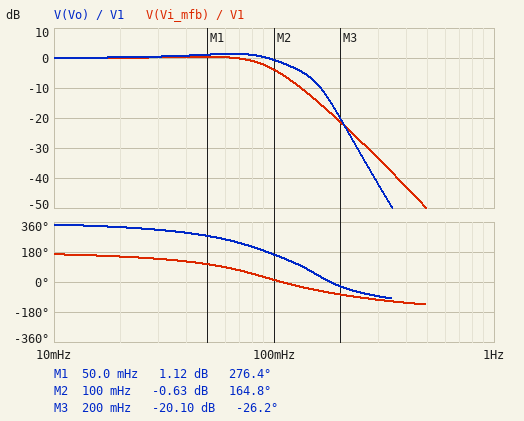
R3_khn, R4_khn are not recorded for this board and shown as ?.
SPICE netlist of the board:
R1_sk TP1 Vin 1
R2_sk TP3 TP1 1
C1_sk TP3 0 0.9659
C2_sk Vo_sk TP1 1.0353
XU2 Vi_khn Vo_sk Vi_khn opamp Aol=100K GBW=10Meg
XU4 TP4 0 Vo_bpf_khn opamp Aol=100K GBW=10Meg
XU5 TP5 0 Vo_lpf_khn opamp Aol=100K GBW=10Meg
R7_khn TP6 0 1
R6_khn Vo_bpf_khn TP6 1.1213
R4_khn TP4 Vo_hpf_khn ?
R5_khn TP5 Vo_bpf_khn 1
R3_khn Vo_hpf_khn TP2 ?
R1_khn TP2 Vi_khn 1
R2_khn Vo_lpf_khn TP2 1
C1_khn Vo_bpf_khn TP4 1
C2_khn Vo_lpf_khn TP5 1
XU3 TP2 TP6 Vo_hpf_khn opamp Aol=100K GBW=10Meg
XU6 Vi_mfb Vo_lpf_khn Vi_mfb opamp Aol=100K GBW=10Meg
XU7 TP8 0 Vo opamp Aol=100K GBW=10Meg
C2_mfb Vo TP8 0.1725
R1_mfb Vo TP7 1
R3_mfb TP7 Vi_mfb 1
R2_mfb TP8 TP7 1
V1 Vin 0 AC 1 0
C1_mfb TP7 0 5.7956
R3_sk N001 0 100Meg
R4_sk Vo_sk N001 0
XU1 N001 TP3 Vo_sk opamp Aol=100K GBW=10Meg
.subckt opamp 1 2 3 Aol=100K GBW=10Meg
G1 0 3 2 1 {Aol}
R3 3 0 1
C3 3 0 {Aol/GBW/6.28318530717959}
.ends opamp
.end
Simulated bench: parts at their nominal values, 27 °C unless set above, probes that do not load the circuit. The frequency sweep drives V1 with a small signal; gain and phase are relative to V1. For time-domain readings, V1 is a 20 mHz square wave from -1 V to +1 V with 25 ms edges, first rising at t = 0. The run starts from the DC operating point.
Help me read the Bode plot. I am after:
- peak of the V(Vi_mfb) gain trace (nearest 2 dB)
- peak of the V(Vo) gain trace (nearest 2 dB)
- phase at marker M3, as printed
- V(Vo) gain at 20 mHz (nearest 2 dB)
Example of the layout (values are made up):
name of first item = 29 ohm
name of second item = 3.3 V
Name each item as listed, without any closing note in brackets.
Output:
peak of the V(Vi_mfb) gain trace = 0 dB
peak of the V(Vo) gain trace = 2 dB
phase at marker M3, as printed = -26.2 deg
V(Vo) gain at 20 mHz = 0 dB
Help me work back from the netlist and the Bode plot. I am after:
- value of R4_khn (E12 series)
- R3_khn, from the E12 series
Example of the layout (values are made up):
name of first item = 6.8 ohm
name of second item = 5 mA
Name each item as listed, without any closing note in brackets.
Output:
value of R4_khn = 1.8 Ω
R3_khn, from the E12 series = 0.56 Ω
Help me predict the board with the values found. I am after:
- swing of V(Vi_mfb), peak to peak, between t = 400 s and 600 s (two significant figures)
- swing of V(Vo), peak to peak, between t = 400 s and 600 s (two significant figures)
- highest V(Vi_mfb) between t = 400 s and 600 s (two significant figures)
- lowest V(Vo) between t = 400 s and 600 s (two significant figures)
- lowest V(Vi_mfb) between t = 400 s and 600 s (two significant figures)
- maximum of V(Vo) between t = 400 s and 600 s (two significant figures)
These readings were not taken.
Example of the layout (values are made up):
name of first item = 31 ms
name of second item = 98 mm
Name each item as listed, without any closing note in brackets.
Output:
swing of V(Vi_mfb), peak to peak, between t = 400 s and 600 s = 2.5 V
swing of V(Vo), peak to peak, between t = 400 s and 600 s = 2.8 V
highest V(Vi_mfb) between t = 400 s and 600 s = 1.2 V
lowest V(Vo) between t = 400 s and 600 s = -1.4 V
lowest V(Vi_mfb) between t = 400 s and 600 s = -1.2 V
maximum of V(Vo) between t = 400 s and 600 s = 1.4 V
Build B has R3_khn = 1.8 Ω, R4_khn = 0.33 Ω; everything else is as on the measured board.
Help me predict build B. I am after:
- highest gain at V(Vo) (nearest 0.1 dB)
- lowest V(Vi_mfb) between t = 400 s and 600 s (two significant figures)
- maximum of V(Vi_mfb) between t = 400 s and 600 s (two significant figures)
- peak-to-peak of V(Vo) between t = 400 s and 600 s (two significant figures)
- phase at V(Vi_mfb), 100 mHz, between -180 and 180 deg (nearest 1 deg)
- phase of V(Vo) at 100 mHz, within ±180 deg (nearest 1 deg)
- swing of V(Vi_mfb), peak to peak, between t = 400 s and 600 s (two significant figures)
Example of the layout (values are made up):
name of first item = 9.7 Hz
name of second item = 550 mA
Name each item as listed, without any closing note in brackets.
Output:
highest gain at V(Vo) = 0 dB
lowest V(Vi_mfb) between t = 400 s and 600 s = -1.0 V
maximum of V(Vi_mfb) between t = 400 s and 600 s = 1.0 V
peak-to-peak of V(Vo) between t = 400 s and 600 s = 2.3 V
phase at V(Vi_mfb), 100 mHz, between -180 and 180 deg = 77 deg
phase of V(Vo) at 100 mHz, within ±180 deg = -131 deg
swing of V(Vi_mfb), peak to peak, between t = 400 s and 600 s = 2.0 V
